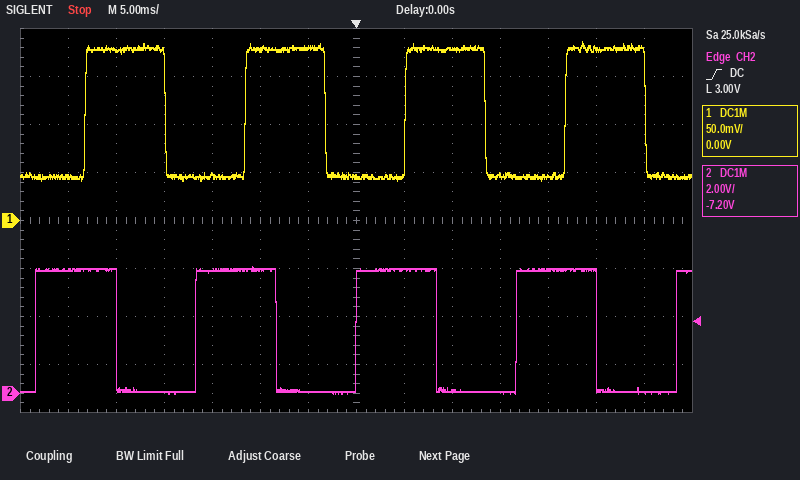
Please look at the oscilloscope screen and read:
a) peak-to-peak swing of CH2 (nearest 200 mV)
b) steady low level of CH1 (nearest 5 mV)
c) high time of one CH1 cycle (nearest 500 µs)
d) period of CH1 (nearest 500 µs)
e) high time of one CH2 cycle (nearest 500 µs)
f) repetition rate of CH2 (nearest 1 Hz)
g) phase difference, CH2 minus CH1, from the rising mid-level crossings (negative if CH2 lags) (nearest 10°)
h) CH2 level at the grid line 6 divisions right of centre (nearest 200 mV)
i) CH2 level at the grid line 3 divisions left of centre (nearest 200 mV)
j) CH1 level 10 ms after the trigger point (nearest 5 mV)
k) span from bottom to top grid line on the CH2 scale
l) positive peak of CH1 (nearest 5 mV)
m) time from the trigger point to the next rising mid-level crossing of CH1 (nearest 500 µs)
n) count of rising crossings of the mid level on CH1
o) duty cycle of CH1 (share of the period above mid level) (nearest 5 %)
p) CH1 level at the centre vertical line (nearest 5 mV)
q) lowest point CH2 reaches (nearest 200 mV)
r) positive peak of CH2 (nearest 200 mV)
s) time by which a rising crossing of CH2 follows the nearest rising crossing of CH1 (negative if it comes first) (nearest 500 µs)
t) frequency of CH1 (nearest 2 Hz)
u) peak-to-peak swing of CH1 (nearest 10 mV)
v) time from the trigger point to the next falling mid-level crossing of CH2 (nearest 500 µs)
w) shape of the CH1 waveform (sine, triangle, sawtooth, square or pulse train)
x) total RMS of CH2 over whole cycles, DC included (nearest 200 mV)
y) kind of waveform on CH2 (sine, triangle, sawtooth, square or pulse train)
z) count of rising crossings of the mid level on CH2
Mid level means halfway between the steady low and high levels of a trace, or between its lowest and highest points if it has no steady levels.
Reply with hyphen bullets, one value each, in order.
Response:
- 5.2 V
- 45 mV
- 8.5 ms
- 16.5 ms
- 8.5 ms
- 60 Hz
- +110°
- 0.0 V
- 5.2 V
- 180 mV
- 16 V
- 185 mV
- 5.0 ms
- 4
- 50 %
- 45 mV
- 0.0 V
- 5.2 V
- -5.0 ms
- 60 Hz
- 140 mV
- 8.5 ms
- square
- 3.6 V
- square
- 5
